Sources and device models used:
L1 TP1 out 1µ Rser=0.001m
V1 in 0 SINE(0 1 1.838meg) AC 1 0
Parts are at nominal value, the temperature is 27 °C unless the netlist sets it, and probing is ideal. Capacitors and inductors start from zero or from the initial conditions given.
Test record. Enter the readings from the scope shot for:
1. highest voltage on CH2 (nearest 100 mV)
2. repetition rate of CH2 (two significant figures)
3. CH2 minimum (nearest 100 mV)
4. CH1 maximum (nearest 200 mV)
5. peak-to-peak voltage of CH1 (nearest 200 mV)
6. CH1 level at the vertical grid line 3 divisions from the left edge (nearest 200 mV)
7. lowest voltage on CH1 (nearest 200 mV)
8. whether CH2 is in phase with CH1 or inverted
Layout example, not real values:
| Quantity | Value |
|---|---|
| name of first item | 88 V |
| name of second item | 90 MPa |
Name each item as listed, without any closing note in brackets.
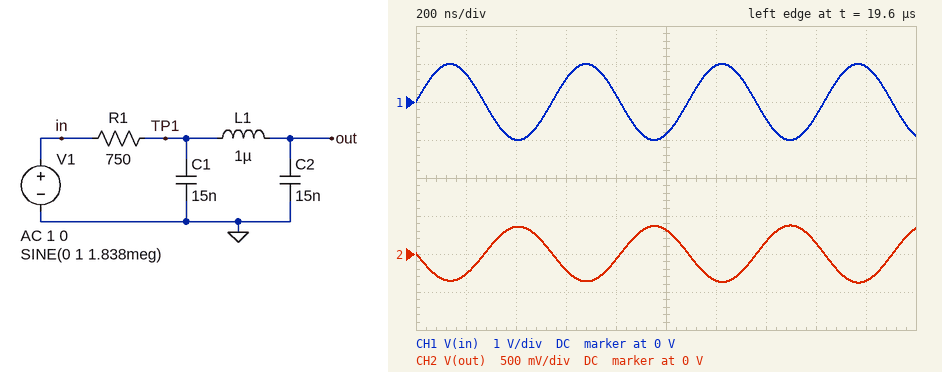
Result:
| Quantity | Value |
|---|---|
| highest voltage on CH2 | 400 mV |
| repetition rate of CH2 | 1.8 MHz |
| CH2 minimum | -400 mV |
| CH1 maximum | 1.0 V |
| peak-to-peak voltage of CH1 | 2.0 V |
| CH1 level at the vertical grid line 3 divisions from the left edge | 600 mV |
| lowest voltage on CH1 | -1.0 V |
| whether CH2 is in phase with CH1 or inverted | inverted |
